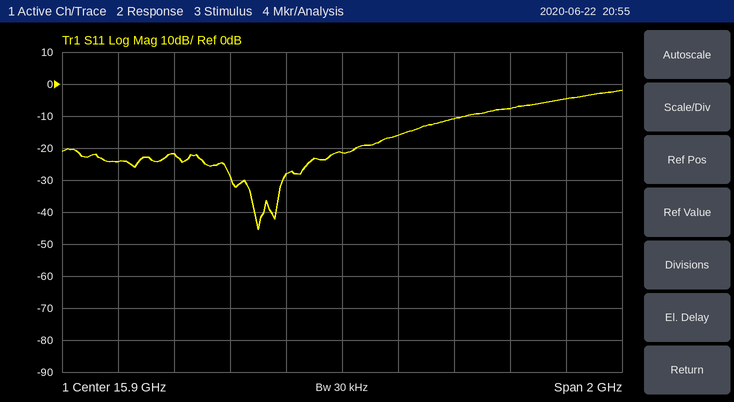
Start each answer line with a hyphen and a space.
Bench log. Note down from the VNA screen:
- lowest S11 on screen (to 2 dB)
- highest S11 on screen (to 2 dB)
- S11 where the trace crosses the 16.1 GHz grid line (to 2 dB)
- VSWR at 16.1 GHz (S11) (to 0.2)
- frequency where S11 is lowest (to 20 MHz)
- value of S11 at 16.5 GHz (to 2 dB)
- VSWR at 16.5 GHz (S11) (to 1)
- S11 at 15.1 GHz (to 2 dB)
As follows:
- -46 dB
- -2 dB
- -16 dB
- 1.4
- 15.60 GHz
- -8 dB
- 2
- -24 dB
